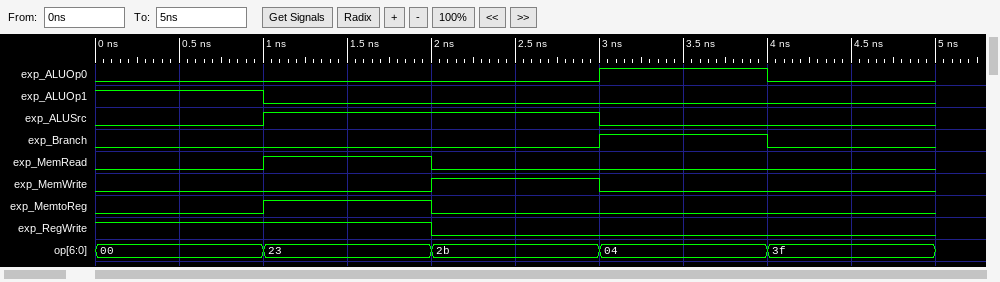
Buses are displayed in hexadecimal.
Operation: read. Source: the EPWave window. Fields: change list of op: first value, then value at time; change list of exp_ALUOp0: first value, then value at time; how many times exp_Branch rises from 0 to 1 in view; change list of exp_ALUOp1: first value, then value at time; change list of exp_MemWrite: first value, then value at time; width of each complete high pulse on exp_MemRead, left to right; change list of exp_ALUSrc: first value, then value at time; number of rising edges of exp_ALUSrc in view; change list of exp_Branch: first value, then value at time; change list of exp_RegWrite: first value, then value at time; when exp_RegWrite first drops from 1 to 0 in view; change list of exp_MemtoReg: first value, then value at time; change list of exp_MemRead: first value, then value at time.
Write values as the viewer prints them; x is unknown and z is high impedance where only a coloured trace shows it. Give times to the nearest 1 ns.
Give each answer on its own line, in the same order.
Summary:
00, 23 at 1 ns, 2b at 2 ns, 04 at 3 ns, 3f at 4 ns
0, 1 at 3 ns, 0 at 4 ns
1
1, 0 at 1 ns
0, 1 at 2 ns, 0 at 3 ns
1 ns
0, 1 at 1 ns, 0 at 3 ns
1
0, 1 at 3 ns, 0 at 4 ns
1, 0 at 2 ns
2 ns
0, 1 at 1 ns, 0 at 2 ns
0, 1 at 1 ns, 0 at 2 ns
